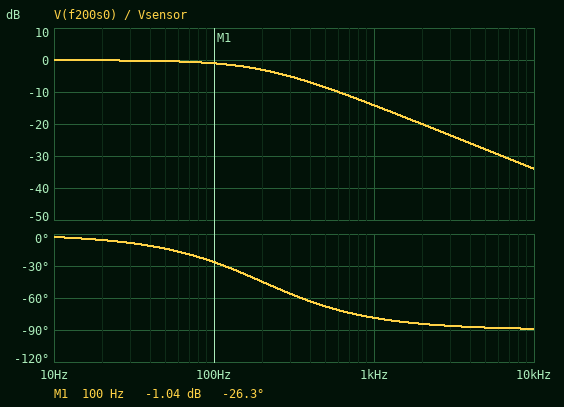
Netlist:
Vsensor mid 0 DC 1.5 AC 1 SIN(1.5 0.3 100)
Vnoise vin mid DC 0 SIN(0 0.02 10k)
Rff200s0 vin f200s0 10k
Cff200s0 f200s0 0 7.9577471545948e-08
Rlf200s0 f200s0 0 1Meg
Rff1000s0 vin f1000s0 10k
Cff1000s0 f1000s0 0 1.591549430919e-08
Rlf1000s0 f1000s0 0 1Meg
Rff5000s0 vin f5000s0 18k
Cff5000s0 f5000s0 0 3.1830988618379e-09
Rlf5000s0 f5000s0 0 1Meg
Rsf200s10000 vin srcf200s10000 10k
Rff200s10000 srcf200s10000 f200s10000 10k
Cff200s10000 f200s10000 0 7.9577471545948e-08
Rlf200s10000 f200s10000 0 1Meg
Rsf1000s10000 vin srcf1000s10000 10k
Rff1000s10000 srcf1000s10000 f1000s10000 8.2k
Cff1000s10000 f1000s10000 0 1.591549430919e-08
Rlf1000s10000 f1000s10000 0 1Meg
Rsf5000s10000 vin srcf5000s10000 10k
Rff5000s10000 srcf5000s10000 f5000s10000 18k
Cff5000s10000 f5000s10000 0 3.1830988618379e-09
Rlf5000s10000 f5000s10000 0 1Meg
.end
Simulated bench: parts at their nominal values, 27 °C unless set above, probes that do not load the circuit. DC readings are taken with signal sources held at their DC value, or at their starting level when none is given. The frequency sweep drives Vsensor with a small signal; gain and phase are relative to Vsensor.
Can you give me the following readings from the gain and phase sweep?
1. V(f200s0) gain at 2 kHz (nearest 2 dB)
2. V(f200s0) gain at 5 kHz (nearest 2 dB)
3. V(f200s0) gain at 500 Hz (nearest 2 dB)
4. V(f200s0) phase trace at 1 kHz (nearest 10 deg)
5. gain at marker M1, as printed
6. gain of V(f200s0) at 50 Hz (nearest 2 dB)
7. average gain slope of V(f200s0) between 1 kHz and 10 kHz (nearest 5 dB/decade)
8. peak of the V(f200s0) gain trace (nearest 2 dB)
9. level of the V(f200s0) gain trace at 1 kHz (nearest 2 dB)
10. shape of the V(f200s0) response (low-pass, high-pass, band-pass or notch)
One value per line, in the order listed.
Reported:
-20 dB
-28 dB
-8 dB
-80 deg
-1.04 dB
0 dB
-20 dB/decade
0 dB
-14 dB
low-pass
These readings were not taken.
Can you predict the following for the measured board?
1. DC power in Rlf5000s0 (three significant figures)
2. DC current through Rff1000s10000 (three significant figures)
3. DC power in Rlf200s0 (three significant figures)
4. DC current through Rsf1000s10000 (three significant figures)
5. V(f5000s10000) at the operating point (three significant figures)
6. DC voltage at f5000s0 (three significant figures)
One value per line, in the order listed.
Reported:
2.17 µW
1.47 µA
2.21 µW
1.47 µA
1.46 V
1.47 V
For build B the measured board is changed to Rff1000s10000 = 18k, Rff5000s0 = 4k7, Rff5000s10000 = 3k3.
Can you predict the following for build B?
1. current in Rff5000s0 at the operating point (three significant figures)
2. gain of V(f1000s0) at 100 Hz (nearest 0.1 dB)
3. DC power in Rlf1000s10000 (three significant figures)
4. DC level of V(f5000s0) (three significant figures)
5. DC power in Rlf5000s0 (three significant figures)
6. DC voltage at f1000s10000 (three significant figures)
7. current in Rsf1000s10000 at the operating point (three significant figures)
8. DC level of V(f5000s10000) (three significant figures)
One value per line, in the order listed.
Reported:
1.49 µA
-0.1 dB
2.13 µW
1.49 V
2.23 µW
1.46 V
1.46 µA
1.48 V
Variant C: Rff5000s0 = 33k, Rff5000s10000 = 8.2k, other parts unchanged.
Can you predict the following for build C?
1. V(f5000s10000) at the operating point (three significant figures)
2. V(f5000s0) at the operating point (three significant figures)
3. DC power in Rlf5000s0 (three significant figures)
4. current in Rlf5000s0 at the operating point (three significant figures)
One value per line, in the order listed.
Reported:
1.47 V
1.45 V
2.11 µW
1.45 µA
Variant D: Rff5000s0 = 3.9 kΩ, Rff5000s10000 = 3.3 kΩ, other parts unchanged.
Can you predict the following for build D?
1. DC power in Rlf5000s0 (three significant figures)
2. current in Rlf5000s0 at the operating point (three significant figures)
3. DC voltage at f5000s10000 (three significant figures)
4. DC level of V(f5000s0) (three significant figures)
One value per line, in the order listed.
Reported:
2.23 µW
1.49 µA
1.48 V
1.49 V
